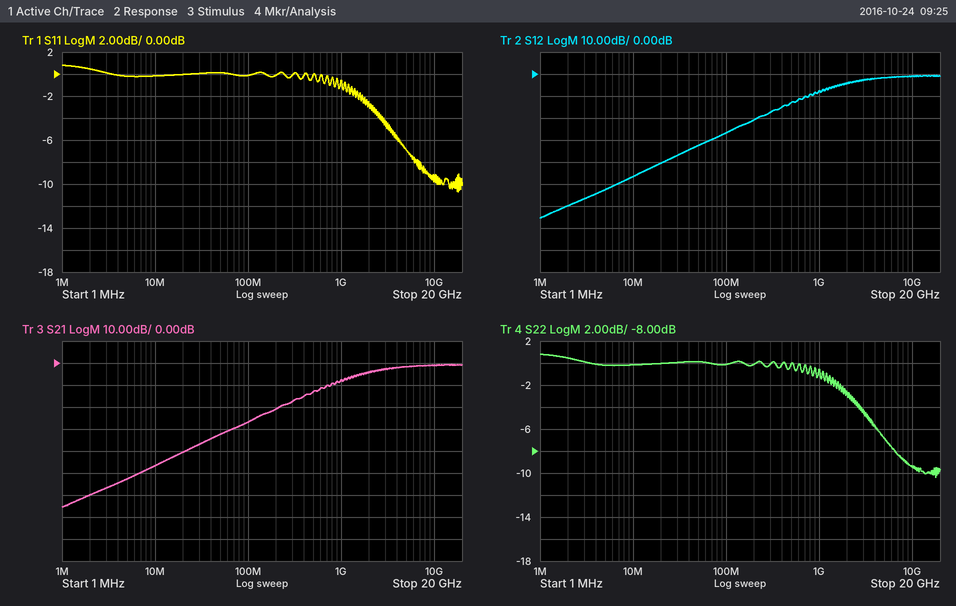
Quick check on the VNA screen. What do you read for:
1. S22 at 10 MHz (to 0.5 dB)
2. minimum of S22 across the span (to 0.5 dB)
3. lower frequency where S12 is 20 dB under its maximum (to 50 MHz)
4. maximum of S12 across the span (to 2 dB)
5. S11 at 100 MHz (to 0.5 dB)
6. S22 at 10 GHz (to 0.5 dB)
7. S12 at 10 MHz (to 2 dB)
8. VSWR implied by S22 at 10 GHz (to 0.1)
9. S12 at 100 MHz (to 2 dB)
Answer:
0.0 dB
-10.5 dB
200 MHz
0 dB
0.0 dB
-9.5 dB
-46 dB
2.0
-26 dB
